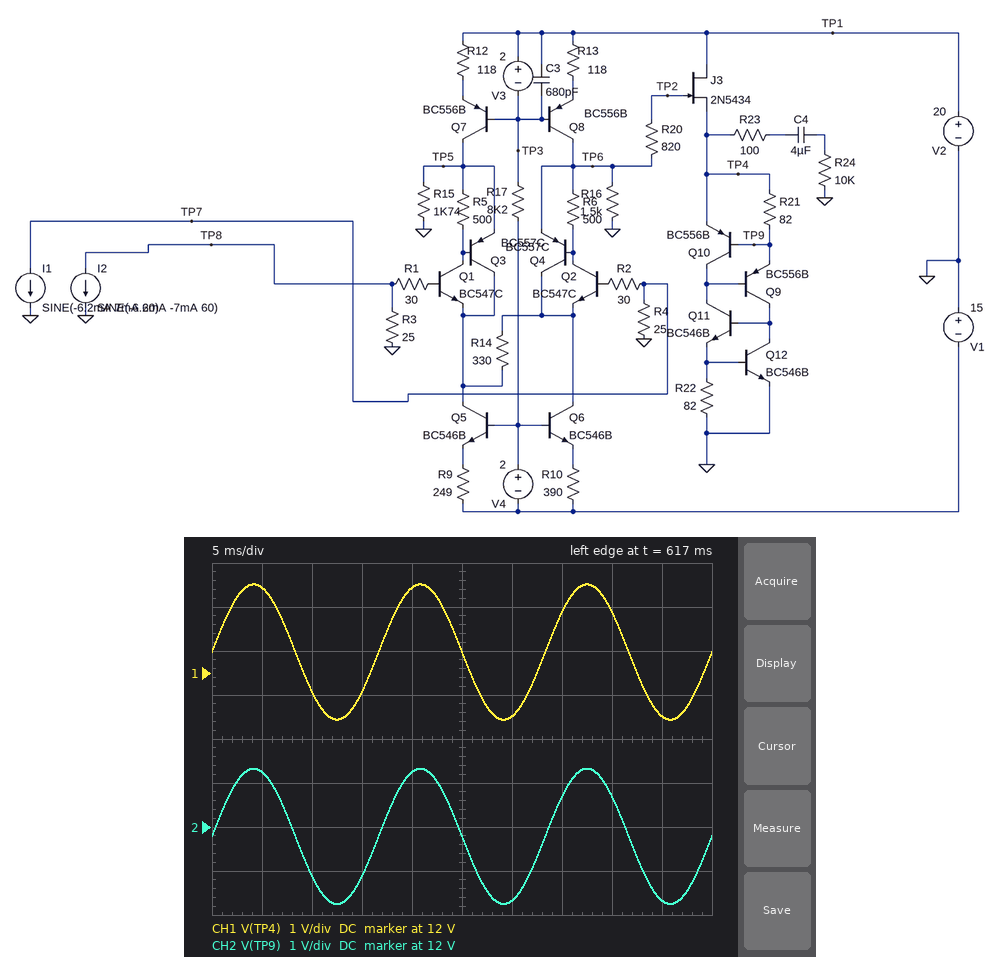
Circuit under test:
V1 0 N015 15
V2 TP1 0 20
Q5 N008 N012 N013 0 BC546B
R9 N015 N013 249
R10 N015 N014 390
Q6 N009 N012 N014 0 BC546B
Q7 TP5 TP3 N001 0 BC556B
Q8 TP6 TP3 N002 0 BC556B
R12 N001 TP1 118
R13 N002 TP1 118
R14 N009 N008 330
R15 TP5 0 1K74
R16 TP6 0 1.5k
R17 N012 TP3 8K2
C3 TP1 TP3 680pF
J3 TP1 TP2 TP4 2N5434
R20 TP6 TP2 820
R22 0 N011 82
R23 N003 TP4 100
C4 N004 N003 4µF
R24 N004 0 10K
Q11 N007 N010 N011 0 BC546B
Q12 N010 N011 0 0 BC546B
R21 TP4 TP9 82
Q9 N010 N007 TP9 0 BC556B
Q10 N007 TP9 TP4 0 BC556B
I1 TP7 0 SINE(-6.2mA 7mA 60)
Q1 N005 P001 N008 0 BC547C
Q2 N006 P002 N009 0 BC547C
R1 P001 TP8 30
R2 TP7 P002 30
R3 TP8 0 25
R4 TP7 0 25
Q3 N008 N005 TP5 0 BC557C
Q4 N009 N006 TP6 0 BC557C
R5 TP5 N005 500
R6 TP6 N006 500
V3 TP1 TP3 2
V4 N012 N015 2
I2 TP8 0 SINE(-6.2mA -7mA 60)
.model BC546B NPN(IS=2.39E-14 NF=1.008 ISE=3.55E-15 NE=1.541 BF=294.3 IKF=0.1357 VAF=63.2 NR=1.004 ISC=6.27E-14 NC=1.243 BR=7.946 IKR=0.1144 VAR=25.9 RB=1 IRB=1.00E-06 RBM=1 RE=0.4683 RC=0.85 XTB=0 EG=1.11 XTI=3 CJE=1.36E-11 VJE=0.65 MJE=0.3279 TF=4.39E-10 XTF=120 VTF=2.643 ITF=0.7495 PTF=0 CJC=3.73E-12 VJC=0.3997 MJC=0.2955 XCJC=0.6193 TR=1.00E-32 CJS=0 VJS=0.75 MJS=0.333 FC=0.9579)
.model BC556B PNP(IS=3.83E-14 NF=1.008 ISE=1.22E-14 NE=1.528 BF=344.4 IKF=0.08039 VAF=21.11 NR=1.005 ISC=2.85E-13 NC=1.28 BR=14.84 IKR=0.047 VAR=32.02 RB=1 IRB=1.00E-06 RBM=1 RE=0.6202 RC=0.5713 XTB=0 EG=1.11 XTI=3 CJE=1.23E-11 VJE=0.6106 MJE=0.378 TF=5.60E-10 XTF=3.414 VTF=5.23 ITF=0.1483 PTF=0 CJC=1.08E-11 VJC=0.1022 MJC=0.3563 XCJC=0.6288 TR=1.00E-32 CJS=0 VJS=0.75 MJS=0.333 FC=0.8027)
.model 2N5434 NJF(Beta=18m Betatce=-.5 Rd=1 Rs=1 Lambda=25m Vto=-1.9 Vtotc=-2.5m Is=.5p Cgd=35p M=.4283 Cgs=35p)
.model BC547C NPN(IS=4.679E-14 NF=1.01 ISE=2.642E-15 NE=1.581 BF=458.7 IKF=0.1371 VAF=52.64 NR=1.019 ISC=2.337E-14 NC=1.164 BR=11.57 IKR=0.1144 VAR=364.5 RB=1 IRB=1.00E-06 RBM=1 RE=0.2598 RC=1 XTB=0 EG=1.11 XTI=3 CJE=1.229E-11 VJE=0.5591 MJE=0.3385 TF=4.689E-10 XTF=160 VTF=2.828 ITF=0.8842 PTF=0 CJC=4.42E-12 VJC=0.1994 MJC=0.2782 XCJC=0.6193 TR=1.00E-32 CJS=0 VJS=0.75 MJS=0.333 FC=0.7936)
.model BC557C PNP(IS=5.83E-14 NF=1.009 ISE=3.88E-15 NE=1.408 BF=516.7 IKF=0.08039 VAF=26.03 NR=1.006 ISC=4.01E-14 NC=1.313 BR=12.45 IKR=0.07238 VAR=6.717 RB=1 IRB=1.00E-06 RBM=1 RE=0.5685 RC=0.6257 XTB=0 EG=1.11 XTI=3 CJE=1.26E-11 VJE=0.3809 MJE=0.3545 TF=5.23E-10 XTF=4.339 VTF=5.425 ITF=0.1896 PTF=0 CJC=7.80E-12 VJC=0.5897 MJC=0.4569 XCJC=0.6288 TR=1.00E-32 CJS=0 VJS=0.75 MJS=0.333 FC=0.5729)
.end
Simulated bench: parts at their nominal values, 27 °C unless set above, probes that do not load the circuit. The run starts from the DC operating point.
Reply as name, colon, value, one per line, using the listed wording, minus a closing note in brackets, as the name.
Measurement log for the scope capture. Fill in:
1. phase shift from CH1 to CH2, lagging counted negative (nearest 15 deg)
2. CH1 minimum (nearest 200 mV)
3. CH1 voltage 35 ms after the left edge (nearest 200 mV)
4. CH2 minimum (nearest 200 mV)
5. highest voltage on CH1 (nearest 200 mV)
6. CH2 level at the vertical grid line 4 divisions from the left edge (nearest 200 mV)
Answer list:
phase shift from CH1 to CH2, lagging counted negative: 0 deg
CH1 minimum: 11.0 V
CH1 voltage 35 ms after the left edge: 13.4 V
CH2 minimum: 10.2 V
highest voltage on CH1: 14.0 V
CH2 level at the vertical grid line 4 divisions from the left edge: 13.2 V
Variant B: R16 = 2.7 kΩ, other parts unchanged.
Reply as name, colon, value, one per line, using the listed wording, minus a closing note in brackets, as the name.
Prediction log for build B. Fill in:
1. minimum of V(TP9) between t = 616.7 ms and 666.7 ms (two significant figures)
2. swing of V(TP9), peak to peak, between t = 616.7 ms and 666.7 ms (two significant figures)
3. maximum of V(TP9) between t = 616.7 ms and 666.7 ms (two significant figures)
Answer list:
minimum of V(TP9) between t = 616.7 ms and 666.7 ms: 18 V
swing of V(TP9), peak to peak, between t = 616.7 ms and 666.7 ms: 890 mV
maximum of V(TP9) between t = 616.7 ms and 666.7 ms: 19 V
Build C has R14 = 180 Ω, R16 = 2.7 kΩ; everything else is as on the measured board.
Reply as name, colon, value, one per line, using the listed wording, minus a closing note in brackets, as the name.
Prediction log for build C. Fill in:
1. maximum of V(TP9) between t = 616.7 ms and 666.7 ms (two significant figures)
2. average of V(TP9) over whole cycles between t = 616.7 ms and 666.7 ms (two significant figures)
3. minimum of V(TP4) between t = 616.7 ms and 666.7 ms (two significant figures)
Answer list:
maximum of V(TP9) between t = 616.7 ms and 666.7 ms: 19 V
average of V(TP9) over whole cycles between t = 616.7 ms and 666.7 ms: 18 V
minimum of V(TP4) between t = 616.7 ms and 666.7 ms: 16 V
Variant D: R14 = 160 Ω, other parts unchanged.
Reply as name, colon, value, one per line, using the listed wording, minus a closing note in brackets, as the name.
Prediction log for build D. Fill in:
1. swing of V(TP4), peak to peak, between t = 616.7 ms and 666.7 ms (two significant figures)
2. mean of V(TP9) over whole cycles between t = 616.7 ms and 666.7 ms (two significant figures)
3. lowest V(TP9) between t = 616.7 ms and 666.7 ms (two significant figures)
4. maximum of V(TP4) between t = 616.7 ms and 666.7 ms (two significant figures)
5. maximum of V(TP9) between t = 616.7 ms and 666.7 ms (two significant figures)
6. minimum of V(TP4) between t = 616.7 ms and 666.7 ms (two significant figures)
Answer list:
swing of V(TP4), peak to peak, between t = 616.7 ms and 666.7 ms: 6.3 V
mean of V(TP9) over whole cycles between t = 616.7 ms and 666.7 ms: 12 V
lowest V(TP9) between t = 616.7 ms and 666.7 ms: 8.6 V
maximum of V(TP4) between t = 616.7 ms and 666.7 ms: 16 V
maximum of V(TP9) between t = 616.7 ms and 666.7 ms: 15 V
minimum of V(TP4) between t = 616.7 ms and 666.7 ms: 9.3 V
